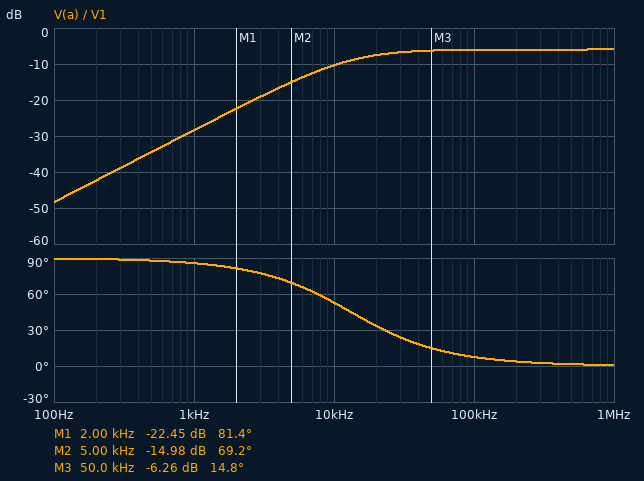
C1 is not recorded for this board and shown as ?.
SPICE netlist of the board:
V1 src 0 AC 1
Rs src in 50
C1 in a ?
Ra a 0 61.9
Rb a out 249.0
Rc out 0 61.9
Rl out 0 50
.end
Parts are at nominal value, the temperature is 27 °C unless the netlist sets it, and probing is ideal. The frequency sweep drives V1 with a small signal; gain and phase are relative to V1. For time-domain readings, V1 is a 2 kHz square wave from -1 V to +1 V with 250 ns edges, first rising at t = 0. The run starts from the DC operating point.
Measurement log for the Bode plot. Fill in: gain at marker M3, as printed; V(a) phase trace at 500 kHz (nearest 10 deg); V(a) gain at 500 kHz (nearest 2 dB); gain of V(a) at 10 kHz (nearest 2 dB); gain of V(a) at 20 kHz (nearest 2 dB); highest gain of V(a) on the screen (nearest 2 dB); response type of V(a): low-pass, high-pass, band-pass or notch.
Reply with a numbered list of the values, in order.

1. -6.26 dB
2. 0 deg
3. -6 dB
4. -10 dB
5. -8 dB
6. -6 dB
7. high-pass
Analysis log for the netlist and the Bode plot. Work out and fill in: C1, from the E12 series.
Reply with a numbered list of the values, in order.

1. 120 nF
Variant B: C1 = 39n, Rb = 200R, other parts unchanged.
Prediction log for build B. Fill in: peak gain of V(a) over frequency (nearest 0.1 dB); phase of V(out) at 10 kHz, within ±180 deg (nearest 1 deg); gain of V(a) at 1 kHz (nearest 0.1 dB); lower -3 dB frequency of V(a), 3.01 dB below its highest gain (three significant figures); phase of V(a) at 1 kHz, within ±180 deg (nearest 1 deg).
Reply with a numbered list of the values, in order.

1. -6.1 dB
2. 76 deg
3. -38.5 dB
4. 41.4 kHz
5. 89 deg
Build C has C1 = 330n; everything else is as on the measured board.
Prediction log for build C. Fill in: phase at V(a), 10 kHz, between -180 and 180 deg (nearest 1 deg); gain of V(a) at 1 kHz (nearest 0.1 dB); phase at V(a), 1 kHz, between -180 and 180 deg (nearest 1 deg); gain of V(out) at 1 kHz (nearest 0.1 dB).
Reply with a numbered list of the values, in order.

1. 26 deg
2. -19.8 dB
3. 78 deg
4. -39.8 dB
